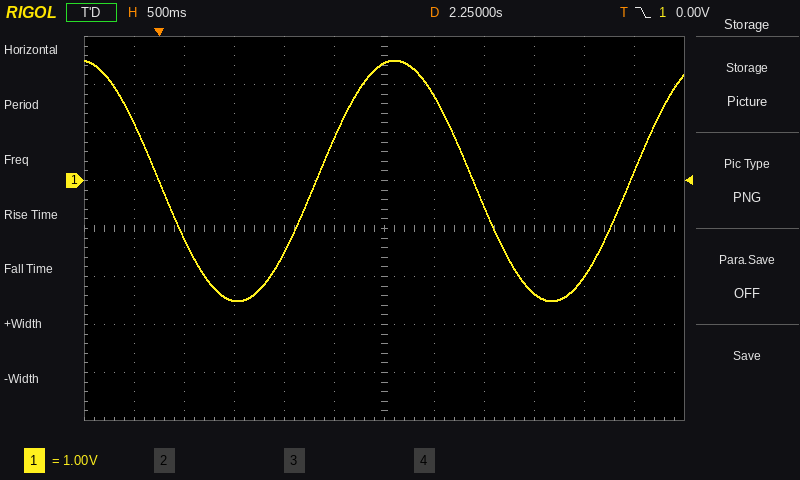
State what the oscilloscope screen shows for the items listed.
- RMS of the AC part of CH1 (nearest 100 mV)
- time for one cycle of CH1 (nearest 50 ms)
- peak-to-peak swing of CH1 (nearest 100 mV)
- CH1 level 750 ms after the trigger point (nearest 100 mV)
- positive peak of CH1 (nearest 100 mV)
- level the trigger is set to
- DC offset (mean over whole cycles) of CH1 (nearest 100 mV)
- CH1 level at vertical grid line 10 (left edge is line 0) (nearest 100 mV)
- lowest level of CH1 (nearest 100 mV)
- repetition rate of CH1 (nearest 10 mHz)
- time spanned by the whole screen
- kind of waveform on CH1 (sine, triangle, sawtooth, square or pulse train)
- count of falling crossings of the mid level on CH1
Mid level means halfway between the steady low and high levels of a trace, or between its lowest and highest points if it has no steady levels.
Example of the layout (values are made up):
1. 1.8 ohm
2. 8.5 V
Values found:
1. 1.8 V
2. 3.15 s
3. 5.0 V
4. -2.5 V
5. 2.5 V
6. 0.00 V
7. 0.0 V
8. -2.0 V
9. -2.5 V
10. 320 mHz
11. 6 s
12. sine
13. 2
